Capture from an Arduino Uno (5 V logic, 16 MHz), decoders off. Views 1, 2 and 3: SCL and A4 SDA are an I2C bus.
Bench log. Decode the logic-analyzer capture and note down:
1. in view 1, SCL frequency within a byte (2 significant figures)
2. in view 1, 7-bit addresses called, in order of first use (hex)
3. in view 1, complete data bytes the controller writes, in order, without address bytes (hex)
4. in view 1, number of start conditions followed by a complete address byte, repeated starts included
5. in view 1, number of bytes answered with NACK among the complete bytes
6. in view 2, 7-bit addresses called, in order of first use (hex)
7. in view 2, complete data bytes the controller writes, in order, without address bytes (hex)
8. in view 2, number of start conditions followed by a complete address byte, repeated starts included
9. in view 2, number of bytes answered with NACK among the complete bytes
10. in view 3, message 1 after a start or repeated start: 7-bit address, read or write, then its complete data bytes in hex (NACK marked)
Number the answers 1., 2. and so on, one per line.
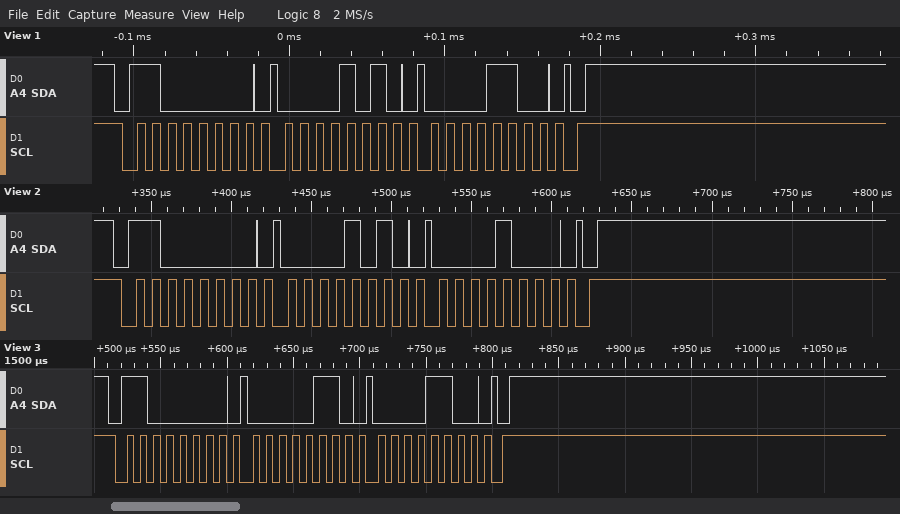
1. 100 kHz
2. 0x60
3. 0A 0C
4. 1
5. 0
6. 0x60
7. 0A 08
8. 1
9. 0
10. 0x60 write: 06 0C
